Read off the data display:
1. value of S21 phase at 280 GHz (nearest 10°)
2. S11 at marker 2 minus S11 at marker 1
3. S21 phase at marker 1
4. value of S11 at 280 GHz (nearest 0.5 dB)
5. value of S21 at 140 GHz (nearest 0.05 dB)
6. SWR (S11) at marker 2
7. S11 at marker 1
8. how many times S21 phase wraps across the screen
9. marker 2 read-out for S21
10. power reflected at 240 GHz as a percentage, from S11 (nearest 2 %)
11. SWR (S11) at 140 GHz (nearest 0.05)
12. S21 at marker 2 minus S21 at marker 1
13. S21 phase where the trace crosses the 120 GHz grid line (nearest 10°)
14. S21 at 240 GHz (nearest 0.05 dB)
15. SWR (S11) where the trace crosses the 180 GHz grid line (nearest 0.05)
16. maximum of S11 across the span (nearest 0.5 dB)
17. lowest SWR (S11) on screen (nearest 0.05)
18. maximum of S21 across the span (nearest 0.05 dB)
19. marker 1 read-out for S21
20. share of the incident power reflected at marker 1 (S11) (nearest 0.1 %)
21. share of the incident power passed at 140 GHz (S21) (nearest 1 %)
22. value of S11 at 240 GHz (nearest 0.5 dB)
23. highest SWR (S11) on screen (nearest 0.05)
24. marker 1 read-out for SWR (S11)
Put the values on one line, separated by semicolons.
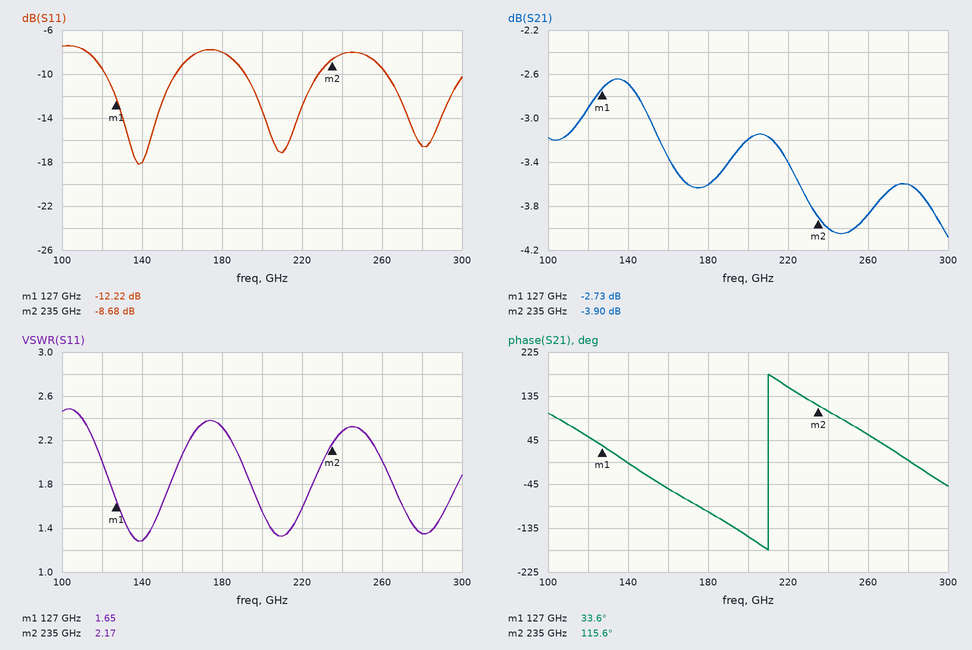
0°; 3.54 dB; 33.6°; -16.5 dB; -2.70 dB; 2.17; -12.22 dB; 1; -3.90 dB; 16 %; 1.30; -1.17 dB; 50°; -4.00 dB; 2.30; -7.5 dB; 1.30; -2.65 dB; -2.73 dB; 6.0 %; 54 %; -8.0 dB; 2.50; 1.65
